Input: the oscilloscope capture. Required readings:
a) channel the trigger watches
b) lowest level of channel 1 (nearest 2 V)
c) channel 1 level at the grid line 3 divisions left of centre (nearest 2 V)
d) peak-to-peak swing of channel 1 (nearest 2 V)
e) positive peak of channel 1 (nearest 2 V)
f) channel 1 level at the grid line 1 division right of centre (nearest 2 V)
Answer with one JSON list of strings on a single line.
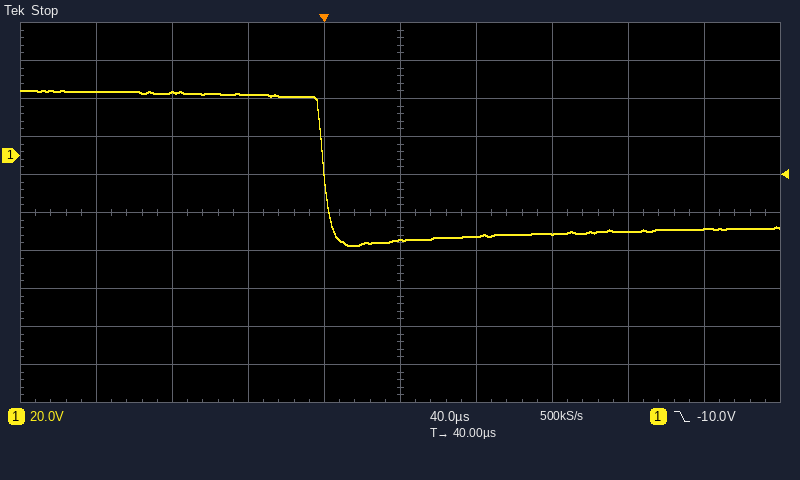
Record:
["channel 1", "-48 V", "34 V", "82 V", "34 V", "-42 V"]
